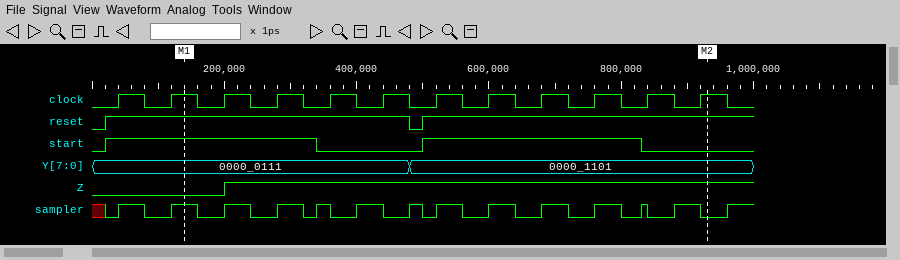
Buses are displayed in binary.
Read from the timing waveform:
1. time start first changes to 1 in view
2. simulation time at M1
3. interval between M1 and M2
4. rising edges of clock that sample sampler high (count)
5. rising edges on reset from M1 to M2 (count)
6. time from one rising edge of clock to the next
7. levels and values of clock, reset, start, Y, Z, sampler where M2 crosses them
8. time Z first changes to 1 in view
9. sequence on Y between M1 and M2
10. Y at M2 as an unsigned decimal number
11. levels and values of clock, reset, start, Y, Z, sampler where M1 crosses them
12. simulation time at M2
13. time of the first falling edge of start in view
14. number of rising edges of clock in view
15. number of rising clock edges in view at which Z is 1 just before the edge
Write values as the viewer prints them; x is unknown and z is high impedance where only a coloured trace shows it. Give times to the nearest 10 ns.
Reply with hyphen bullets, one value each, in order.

- 20 ns
- 140 ns
- 790 ns
- 4
- 1
- 80 ns
- clock=1, reset=1, start=0, Y=0000_1101, Z=1, sampler=0
- 200 ns
- 0000_0111, 0000_1101
- 13
- clock=1, reset=1, start=1, Y=0000_0111, Z=0, sampler=1
- 930 ns
- 340 ns
- 12
- 9
